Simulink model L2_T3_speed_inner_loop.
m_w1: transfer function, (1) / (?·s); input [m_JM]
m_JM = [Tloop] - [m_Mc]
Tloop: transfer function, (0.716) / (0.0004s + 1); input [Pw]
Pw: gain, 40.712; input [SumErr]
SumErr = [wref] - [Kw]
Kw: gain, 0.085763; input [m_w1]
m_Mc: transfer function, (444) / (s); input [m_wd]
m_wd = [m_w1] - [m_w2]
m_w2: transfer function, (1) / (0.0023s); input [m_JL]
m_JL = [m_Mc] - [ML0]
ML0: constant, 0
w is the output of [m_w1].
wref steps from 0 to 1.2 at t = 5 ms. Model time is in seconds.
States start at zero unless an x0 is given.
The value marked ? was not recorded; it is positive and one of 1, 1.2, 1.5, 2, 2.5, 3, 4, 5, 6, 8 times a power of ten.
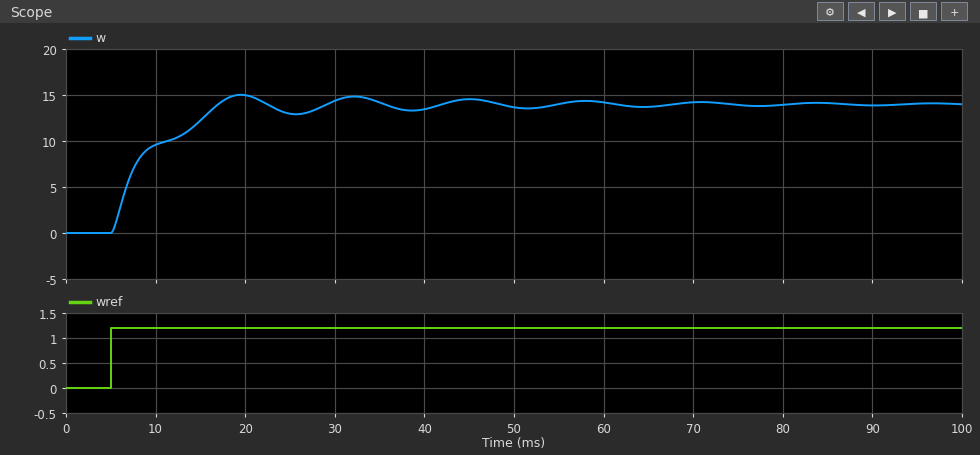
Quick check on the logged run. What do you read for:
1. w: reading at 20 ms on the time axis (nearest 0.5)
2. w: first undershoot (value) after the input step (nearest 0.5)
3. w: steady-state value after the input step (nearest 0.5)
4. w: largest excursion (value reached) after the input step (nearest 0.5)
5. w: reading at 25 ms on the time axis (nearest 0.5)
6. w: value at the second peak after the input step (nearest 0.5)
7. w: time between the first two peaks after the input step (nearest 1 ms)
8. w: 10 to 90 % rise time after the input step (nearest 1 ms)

15.0
13.0
14.0
15.0
13.0
15.0
13 ms
10 ms
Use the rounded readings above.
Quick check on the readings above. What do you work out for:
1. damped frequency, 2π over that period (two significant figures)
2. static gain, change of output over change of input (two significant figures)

0.48 rad/ms
12
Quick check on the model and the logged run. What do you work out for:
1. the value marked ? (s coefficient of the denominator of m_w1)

0.008
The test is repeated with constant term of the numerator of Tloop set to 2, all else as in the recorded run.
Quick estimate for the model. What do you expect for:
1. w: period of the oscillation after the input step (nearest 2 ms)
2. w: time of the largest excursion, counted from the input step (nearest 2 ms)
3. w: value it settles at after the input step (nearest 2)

14 ms
12 ms
14
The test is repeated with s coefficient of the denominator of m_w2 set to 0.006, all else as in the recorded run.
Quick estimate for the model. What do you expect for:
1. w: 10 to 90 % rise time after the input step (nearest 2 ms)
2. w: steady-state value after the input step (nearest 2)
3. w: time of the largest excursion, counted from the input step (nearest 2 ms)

14 ms
14
20 ms
